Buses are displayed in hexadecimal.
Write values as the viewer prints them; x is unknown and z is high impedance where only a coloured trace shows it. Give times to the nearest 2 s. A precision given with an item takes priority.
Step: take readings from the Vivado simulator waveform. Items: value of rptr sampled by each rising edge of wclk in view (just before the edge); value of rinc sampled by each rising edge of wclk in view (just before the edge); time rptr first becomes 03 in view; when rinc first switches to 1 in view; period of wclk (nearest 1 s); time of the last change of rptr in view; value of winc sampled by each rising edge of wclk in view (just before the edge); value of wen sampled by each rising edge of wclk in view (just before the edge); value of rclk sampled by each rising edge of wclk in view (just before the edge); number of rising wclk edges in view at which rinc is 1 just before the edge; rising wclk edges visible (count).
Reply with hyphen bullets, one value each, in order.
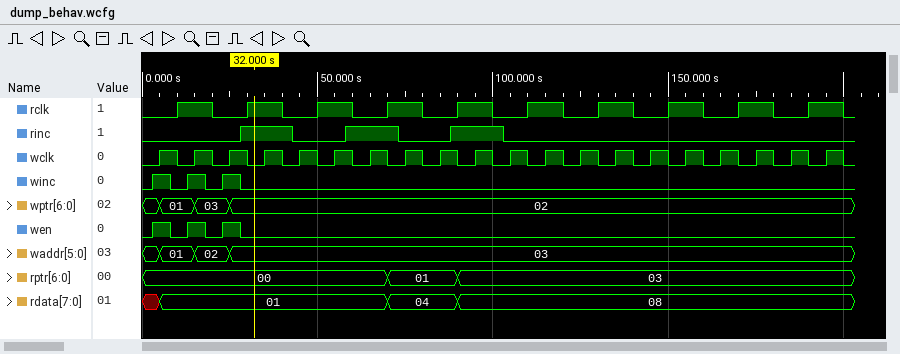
- 00, 00, 00, 00, 00, 00, 00, 01, 01, 03, 03, 03, 03, 03, 03, 03, 03, 03, 03, 03
- 0 0 0 1 0 0 1 0 0 1 0 0 0 0 0 0 0 0 0 0
- 90 s
- 28 s
- 10 s
- 90 s
- 1 1 1 0 0 0 0 0 0 0 0 0 0 0 0 0 0 0 0 0
- 1 1 1 0 0 0 0 0 0 0 0 0 0 0 0 0 0 0 0 0
- 0 1 0 1 0 1 0 1 0 1 0 1 0 1 0 1 0 1 0 1
- 3
- 20
